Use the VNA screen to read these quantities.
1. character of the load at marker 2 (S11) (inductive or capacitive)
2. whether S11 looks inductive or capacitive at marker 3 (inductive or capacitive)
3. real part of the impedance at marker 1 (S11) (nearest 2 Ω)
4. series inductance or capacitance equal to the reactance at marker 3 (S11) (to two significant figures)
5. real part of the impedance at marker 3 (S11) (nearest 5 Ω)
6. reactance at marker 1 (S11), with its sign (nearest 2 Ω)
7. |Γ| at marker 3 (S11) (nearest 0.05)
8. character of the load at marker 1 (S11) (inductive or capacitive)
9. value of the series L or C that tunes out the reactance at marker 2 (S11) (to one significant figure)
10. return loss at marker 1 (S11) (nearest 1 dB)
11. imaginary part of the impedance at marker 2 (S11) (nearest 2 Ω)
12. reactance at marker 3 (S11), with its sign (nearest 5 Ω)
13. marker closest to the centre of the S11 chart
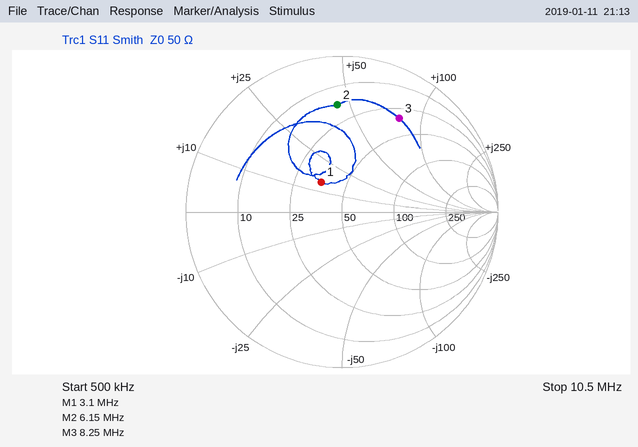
inductive
inductive
36 Ω
1.5 µH
35 Ω
+14 Ω
0.70
inductive
600 pF
13 dB
+44 Ω
+80 Ω
marker 1
